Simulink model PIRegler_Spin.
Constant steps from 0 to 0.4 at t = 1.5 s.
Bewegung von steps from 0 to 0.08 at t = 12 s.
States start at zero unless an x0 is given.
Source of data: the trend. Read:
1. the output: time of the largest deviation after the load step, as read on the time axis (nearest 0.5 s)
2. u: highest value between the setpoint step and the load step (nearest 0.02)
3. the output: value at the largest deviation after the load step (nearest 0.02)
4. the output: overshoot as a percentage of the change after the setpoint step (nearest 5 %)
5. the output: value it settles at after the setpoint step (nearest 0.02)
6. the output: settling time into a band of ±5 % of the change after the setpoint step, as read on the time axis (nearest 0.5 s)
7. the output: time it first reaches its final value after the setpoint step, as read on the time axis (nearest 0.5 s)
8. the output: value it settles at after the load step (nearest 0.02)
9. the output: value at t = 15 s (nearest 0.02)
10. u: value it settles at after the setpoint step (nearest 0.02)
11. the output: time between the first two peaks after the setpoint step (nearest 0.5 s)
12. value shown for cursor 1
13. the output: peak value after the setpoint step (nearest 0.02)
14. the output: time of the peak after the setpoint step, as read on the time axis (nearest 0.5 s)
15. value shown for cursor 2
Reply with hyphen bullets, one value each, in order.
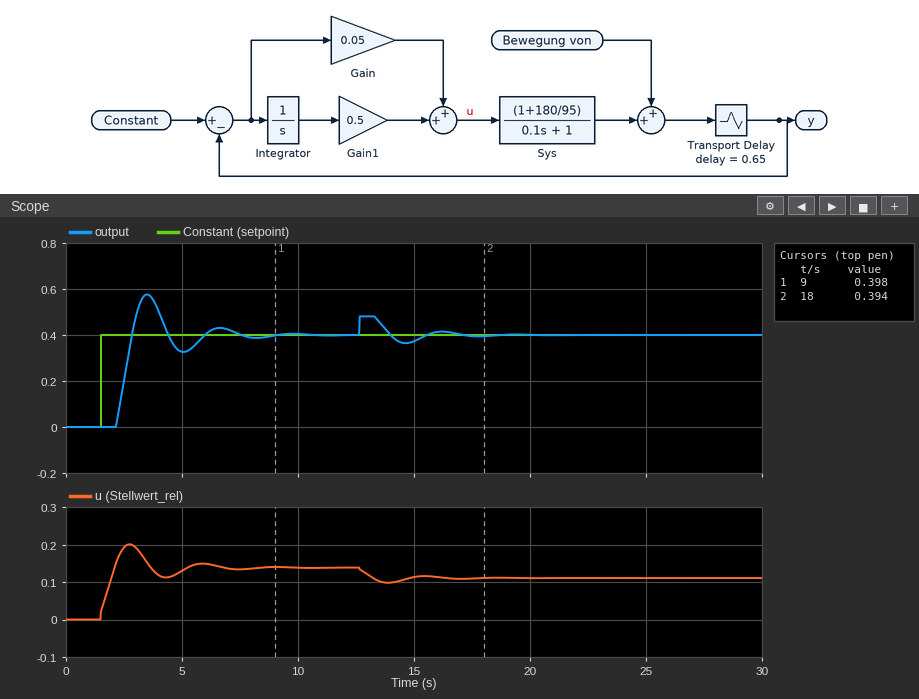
- 13.0 s
- 0.20
- 0.48
- 45 %
- 0.40
- 7.0 s
- 3.0 s
- 0.40
- 0.38
- 0.14
- 3.0 s
- 0.398
- 0.58
- 3.5 s
- 0.394
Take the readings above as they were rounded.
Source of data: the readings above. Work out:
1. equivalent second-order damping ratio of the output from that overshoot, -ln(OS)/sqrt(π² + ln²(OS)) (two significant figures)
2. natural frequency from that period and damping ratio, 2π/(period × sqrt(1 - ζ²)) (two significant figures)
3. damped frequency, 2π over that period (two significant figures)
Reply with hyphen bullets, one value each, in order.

- 0.25
- 2.2 rad/s
- 2.1 rad/s
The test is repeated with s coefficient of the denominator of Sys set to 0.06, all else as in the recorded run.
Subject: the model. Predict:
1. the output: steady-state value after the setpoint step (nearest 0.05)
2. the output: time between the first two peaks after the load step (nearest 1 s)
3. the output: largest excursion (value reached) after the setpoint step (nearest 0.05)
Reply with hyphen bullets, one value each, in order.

- 0.40
- 3 s
- 0.55
